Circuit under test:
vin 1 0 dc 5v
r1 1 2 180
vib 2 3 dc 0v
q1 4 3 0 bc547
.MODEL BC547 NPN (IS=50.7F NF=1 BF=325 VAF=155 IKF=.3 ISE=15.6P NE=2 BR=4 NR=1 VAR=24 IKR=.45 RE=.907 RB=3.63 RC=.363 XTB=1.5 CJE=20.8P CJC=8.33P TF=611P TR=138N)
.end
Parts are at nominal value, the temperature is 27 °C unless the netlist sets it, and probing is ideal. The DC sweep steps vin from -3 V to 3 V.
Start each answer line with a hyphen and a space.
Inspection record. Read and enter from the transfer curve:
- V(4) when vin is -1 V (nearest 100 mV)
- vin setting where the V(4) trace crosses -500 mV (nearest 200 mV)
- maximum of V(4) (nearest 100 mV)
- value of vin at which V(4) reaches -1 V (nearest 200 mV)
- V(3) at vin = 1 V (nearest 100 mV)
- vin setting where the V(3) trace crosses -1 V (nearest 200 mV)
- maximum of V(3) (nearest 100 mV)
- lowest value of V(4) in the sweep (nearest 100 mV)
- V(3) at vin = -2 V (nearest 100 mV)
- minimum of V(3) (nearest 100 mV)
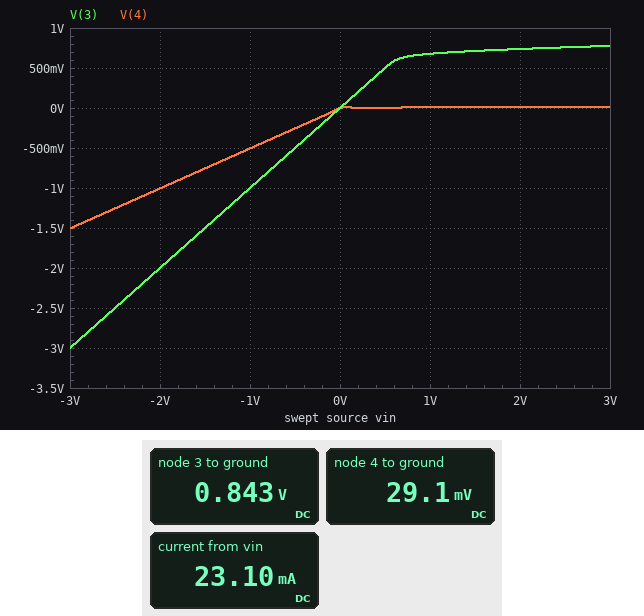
- -500 mV
- -1.0 V
- 0 V
- -2.0 V
- 700 mV
- -1.0 V
- 800 mV
- -1.5 V
- -2.0 V
- -3.0 V
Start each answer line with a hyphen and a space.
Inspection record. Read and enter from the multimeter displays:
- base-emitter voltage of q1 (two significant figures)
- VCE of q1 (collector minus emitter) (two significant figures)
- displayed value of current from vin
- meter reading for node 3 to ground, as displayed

- 840 mV
- 29 mV
- 23.10 mA
- 0.843 V
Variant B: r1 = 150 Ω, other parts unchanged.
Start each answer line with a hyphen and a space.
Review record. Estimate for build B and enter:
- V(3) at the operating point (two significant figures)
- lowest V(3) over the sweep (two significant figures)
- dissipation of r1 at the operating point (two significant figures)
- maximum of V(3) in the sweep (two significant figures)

- 870 mV
- -3.0 V
- 110 mW
- 790 mV
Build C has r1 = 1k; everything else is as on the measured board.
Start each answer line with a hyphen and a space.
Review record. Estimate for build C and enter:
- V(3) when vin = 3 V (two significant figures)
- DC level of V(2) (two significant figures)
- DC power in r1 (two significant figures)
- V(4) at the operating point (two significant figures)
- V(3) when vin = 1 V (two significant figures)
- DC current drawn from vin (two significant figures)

- 690 mV
- 710 mV
- 18 mW
- 10 mV
- 630 mV
- 4.3 mA
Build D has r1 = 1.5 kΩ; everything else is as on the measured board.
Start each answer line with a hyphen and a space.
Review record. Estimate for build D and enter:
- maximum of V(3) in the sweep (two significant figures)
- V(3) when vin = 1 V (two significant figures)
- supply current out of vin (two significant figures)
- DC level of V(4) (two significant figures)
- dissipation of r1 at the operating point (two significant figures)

- 670 mV
- 620 mV
- 2.9 mA
- 8.9 mV
- 12 mW
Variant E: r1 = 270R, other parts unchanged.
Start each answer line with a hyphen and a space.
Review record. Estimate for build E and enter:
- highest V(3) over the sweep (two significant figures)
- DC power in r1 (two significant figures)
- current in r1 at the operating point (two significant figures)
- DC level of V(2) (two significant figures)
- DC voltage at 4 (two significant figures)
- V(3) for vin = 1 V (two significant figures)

- 750 mV
- 65 mW
- 16 mA
- 800 mV
- 22 mV
- 670 mV
